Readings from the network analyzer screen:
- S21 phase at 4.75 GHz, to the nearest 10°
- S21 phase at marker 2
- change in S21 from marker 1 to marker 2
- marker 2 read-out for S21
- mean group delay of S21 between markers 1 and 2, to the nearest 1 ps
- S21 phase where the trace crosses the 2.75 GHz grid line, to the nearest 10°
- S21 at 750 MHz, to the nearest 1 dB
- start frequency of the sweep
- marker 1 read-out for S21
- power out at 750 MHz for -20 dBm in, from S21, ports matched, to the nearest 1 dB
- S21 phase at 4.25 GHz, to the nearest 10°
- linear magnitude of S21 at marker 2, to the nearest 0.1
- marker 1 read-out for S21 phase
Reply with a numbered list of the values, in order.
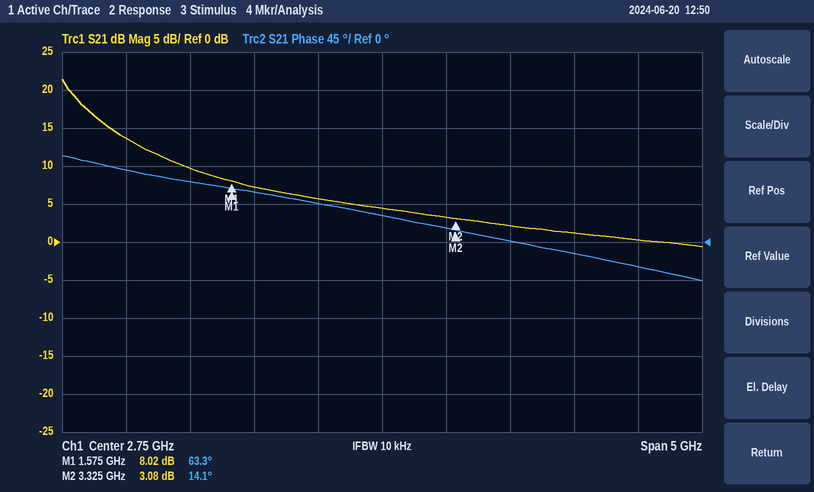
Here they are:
1. -30°
2. 14.1°
3. -4.94 dB
4. 3.08 dB
5. 78 ps
6. 30°
7. 14 dB
8. 250 MHz
9. 8.02 dB
10. -6 dBm
11. -10°
12. 1.4
13. 63.3°
